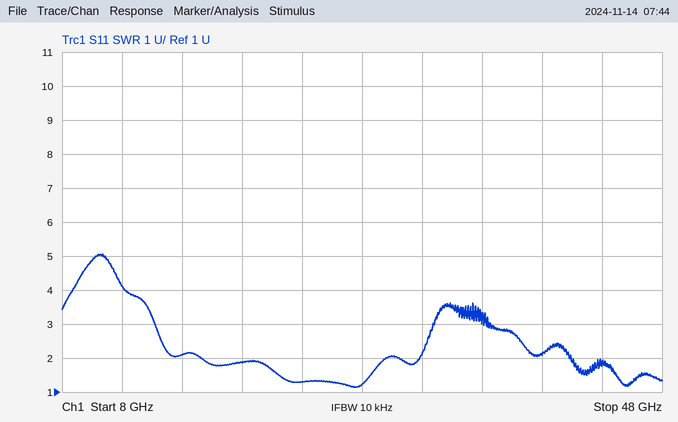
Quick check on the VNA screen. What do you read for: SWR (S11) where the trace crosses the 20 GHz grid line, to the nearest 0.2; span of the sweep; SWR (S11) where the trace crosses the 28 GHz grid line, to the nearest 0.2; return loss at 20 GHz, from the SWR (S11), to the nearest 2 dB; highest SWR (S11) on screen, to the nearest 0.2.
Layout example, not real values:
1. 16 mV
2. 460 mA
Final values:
1. 1.8
2. 40 GHz
3. 1.2
4. 10 dB
5. 5.0
